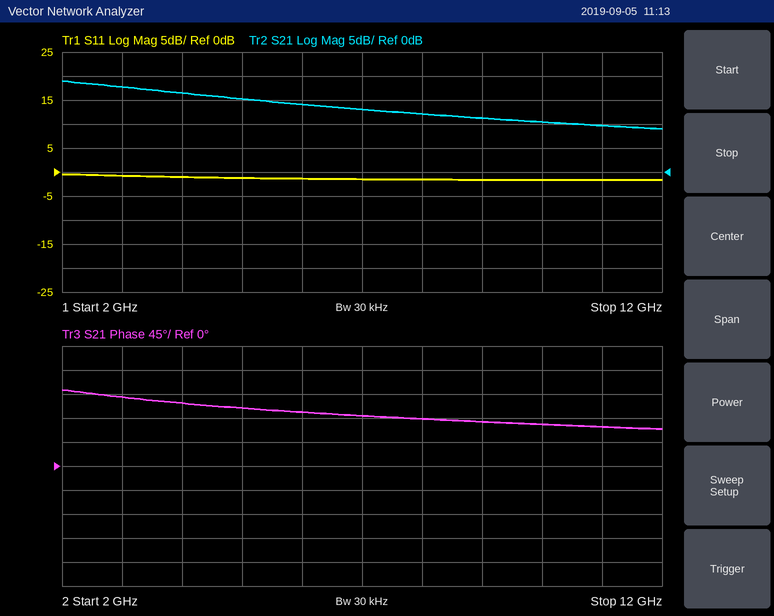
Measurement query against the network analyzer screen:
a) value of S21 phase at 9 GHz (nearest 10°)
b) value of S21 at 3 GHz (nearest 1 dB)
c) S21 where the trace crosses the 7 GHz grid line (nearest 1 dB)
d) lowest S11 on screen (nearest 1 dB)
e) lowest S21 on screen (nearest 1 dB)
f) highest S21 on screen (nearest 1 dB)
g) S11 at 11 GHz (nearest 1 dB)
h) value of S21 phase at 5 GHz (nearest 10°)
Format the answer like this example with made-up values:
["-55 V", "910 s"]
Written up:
["80°", "18 dB", "13 dB", "-2 dB", "9 dB", "19 dB", "-2 dB", "110°"]
